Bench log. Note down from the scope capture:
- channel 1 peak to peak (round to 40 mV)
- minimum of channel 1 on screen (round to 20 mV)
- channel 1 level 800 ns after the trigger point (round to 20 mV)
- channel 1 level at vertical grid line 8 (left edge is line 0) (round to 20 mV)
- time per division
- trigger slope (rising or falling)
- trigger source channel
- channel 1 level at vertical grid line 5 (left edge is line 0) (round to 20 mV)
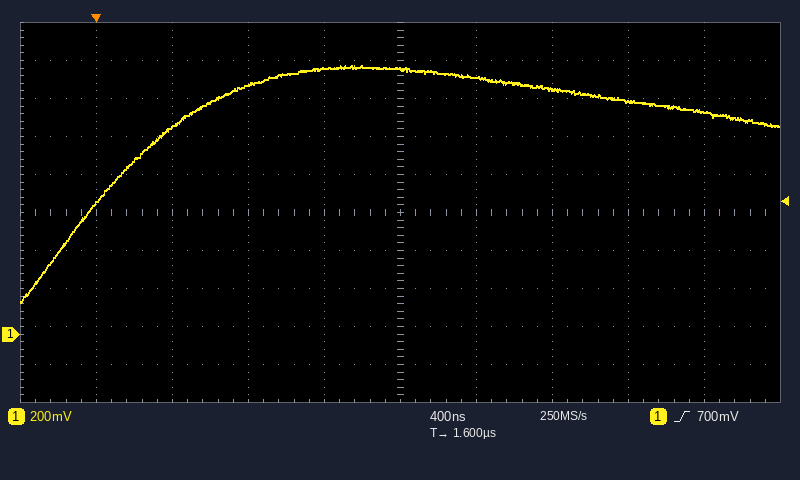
1.24 V
160 mV
1.32 V
1.22 V
400 ns
rising
channel 1
1.40 V
